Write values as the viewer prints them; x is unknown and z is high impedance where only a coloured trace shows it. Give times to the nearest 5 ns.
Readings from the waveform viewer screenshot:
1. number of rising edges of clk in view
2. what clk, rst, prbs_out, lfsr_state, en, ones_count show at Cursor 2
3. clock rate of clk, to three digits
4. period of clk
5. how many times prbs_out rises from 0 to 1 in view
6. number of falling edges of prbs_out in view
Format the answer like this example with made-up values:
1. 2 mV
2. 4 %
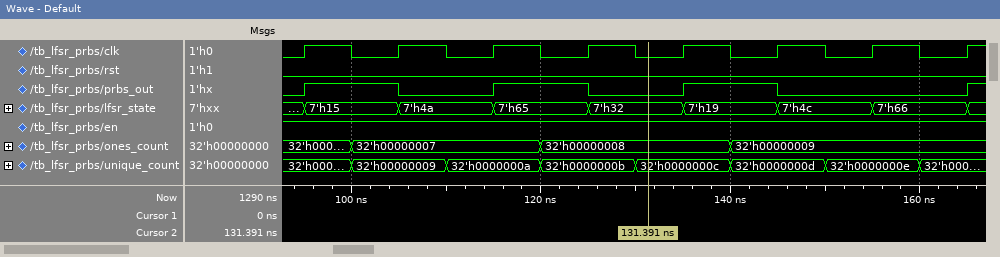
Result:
1. 8
2. clk=0, rst=0, prbs_out=0, lfsr_state=7'h32, en=1, ones_count=32'h00000008
3. 100 MHz
4. 10 ns
5. 4
6. 3
